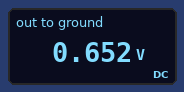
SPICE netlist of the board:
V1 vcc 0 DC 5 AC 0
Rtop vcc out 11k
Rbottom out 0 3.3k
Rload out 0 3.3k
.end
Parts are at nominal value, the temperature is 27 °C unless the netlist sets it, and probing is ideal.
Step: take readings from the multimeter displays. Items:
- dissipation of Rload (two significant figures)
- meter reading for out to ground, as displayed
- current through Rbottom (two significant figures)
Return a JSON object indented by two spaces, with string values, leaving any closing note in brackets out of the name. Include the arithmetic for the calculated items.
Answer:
{
  "dissipation of Rload": "(652 mV)^2 / 3.3 kΩ = 130 µW",
  "meter reading for out to ground, as displayed": "0.652 V",
  "current through Rbottom": "(652 mV) / 3.3 kΩ = 200 µA"
}
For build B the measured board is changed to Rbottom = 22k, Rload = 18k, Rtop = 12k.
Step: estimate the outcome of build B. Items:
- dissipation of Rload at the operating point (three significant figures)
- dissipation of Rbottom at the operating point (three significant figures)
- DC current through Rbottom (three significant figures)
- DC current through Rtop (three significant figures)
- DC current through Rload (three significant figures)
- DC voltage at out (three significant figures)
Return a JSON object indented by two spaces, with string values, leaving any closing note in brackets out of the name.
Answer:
{
  "dissipation of Rload at the operating point": "284 µW",
  "dissipation of Rbottom at the operating point": "232 µW",
  "DC current through Rbottom": "103 µA",
  "DC current through Rtop": "228 µA",
  "DC current through Rload": "126 µA",
  "DC voltage at out": "2.26 V"
}
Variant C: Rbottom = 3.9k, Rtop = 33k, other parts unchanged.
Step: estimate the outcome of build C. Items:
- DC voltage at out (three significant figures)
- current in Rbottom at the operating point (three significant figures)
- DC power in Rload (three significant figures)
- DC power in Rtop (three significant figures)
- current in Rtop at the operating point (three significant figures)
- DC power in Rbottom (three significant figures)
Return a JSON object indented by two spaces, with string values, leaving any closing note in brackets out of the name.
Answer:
{
  "DC voltage at out": "257 mV",
  "current in Rbottom at the operating point": "65.9 µA",
  "DC power in Rload": "20.0 µW",
  "DC power in Rtop": "682 µW",
  "current in Rtop at the operating point": "144 µA",
  "DC power in Rbottom": "16.9 µW"
}
